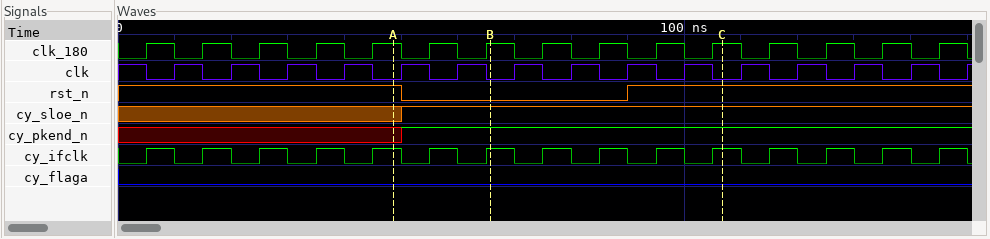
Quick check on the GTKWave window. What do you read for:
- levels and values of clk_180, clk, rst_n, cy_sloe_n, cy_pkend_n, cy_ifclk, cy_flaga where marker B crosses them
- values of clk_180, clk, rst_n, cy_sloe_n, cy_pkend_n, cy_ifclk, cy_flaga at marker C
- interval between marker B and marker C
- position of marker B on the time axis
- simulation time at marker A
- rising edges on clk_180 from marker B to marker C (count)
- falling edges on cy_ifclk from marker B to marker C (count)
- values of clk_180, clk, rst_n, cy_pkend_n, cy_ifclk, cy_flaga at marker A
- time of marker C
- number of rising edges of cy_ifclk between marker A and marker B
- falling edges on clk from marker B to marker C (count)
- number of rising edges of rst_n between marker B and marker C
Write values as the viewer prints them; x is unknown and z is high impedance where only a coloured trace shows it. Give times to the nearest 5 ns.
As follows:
clk_180=1, clk=0, rst_n=0, cy_sloe_n=1, cy_pkend_n=1, cy_ifclk=1, cy_flaga=0
clk_180=1, clk=0, rst_n=1, cy_sloe_n=1, cy_pkend_n=1, cy_ifclk=1, cy_flaga=0
40 ns
65 ns
50 ns
4
4
clk_180=1, clk=0, rst_n=1, cy_pkend_n=x, cy_ifclk=1, cy_flaga=0
105 ns
2
4
1
